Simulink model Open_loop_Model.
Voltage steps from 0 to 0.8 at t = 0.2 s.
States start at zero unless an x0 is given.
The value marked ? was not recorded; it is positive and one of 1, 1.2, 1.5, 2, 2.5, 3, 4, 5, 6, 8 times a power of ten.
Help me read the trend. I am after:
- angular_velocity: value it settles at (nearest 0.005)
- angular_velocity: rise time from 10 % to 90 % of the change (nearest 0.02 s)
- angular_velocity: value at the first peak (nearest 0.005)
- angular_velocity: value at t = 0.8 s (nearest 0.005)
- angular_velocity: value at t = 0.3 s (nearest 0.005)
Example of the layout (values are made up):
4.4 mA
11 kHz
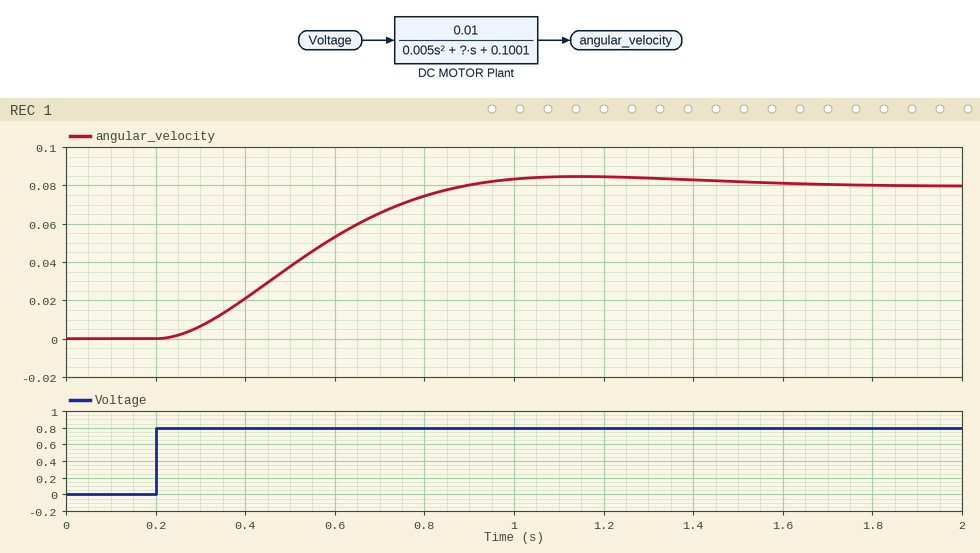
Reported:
0.080
0.46 s
0.085
0.075
0.005
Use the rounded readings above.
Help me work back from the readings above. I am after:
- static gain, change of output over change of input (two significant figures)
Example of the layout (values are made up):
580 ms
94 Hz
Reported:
0.10
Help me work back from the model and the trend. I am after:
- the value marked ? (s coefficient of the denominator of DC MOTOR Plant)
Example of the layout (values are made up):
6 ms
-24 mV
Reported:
0.03
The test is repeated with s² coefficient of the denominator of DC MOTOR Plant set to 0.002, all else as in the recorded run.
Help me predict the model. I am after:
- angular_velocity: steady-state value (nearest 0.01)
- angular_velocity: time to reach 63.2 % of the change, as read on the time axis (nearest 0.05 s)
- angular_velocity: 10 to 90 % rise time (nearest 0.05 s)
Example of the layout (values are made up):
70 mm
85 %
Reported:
0.08
0.50 s
0.50 s
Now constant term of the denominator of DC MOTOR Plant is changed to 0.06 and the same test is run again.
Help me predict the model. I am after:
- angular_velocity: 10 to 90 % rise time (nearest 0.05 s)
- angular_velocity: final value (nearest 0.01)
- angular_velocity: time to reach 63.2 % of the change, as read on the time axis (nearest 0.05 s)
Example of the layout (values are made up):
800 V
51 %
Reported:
0.80 s
0.13
0.75 s
